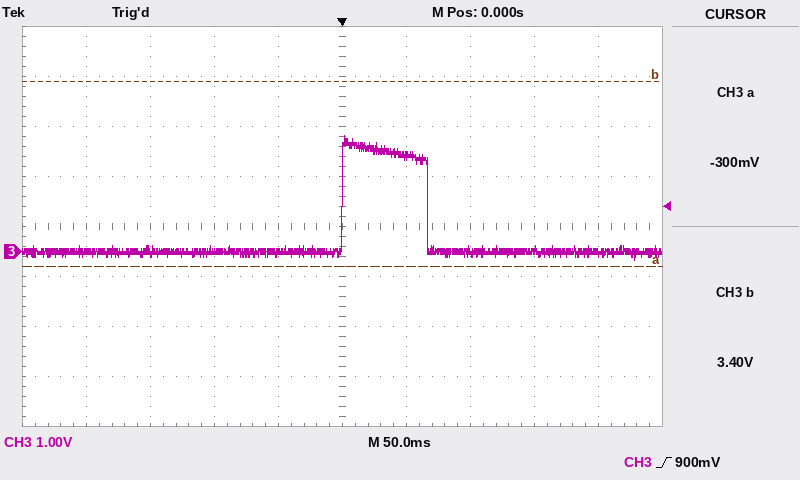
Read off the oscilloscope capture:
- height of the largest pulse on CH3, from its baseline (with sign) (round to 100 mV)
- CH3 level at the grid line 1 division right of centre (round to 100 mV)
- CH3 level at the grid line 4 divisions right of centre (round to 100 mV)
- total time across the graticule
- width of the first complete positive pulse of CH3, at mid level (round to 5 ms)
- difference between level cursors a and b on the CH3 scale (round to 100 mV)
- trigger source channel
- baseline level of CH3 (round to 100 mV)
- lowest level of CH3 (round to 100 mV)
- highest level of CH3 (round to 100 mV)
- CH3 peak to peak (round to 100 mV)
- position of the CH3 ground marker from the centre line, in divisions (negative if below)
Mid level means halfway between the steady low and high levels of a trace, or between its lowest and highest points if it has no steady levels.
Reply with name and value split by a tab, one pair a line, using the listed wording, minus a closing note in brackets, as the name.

height of the largest pulse on CH3, from its baseline (with sign)	+2.3 V
CH3 level at the grid line 1 division right of centre	1.9 V
CH3 level at the grid line 4 divisions right of centre	0.0 V
total time across the graticule	500 ms
width of the first complete positive pulse of CH3, at mid level	65 ms
difference between level cursors a and b on the CH3 scale	3.7 V
trigger source channel	CH3
baseline level of CH3	0.0 V
lowest level of CH3	-200 mV
highest level of CH3	2.3 V
CH3 peak to peak	2.5 V
position of the CH3 ground marker from the centre line, in divisions	-0.5 div
